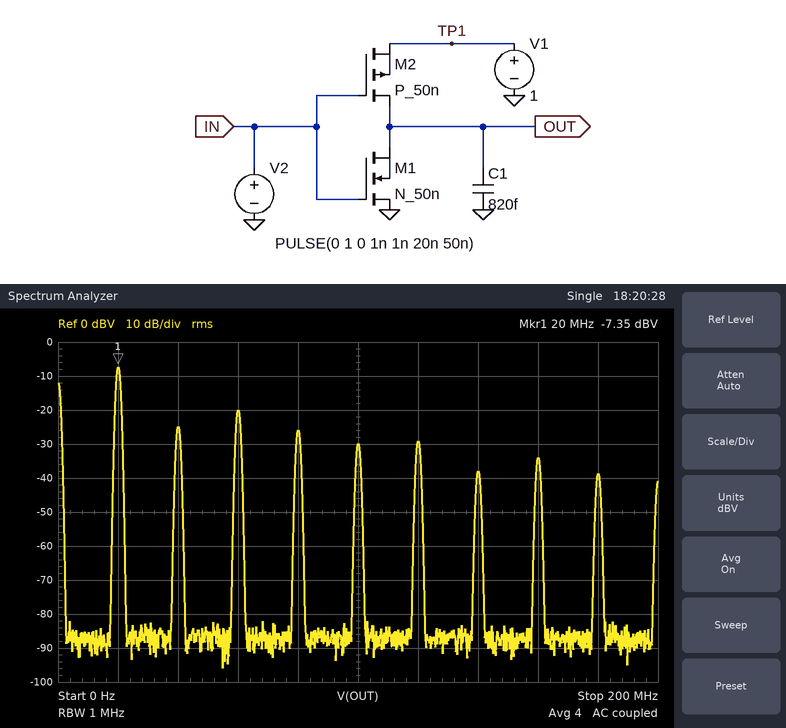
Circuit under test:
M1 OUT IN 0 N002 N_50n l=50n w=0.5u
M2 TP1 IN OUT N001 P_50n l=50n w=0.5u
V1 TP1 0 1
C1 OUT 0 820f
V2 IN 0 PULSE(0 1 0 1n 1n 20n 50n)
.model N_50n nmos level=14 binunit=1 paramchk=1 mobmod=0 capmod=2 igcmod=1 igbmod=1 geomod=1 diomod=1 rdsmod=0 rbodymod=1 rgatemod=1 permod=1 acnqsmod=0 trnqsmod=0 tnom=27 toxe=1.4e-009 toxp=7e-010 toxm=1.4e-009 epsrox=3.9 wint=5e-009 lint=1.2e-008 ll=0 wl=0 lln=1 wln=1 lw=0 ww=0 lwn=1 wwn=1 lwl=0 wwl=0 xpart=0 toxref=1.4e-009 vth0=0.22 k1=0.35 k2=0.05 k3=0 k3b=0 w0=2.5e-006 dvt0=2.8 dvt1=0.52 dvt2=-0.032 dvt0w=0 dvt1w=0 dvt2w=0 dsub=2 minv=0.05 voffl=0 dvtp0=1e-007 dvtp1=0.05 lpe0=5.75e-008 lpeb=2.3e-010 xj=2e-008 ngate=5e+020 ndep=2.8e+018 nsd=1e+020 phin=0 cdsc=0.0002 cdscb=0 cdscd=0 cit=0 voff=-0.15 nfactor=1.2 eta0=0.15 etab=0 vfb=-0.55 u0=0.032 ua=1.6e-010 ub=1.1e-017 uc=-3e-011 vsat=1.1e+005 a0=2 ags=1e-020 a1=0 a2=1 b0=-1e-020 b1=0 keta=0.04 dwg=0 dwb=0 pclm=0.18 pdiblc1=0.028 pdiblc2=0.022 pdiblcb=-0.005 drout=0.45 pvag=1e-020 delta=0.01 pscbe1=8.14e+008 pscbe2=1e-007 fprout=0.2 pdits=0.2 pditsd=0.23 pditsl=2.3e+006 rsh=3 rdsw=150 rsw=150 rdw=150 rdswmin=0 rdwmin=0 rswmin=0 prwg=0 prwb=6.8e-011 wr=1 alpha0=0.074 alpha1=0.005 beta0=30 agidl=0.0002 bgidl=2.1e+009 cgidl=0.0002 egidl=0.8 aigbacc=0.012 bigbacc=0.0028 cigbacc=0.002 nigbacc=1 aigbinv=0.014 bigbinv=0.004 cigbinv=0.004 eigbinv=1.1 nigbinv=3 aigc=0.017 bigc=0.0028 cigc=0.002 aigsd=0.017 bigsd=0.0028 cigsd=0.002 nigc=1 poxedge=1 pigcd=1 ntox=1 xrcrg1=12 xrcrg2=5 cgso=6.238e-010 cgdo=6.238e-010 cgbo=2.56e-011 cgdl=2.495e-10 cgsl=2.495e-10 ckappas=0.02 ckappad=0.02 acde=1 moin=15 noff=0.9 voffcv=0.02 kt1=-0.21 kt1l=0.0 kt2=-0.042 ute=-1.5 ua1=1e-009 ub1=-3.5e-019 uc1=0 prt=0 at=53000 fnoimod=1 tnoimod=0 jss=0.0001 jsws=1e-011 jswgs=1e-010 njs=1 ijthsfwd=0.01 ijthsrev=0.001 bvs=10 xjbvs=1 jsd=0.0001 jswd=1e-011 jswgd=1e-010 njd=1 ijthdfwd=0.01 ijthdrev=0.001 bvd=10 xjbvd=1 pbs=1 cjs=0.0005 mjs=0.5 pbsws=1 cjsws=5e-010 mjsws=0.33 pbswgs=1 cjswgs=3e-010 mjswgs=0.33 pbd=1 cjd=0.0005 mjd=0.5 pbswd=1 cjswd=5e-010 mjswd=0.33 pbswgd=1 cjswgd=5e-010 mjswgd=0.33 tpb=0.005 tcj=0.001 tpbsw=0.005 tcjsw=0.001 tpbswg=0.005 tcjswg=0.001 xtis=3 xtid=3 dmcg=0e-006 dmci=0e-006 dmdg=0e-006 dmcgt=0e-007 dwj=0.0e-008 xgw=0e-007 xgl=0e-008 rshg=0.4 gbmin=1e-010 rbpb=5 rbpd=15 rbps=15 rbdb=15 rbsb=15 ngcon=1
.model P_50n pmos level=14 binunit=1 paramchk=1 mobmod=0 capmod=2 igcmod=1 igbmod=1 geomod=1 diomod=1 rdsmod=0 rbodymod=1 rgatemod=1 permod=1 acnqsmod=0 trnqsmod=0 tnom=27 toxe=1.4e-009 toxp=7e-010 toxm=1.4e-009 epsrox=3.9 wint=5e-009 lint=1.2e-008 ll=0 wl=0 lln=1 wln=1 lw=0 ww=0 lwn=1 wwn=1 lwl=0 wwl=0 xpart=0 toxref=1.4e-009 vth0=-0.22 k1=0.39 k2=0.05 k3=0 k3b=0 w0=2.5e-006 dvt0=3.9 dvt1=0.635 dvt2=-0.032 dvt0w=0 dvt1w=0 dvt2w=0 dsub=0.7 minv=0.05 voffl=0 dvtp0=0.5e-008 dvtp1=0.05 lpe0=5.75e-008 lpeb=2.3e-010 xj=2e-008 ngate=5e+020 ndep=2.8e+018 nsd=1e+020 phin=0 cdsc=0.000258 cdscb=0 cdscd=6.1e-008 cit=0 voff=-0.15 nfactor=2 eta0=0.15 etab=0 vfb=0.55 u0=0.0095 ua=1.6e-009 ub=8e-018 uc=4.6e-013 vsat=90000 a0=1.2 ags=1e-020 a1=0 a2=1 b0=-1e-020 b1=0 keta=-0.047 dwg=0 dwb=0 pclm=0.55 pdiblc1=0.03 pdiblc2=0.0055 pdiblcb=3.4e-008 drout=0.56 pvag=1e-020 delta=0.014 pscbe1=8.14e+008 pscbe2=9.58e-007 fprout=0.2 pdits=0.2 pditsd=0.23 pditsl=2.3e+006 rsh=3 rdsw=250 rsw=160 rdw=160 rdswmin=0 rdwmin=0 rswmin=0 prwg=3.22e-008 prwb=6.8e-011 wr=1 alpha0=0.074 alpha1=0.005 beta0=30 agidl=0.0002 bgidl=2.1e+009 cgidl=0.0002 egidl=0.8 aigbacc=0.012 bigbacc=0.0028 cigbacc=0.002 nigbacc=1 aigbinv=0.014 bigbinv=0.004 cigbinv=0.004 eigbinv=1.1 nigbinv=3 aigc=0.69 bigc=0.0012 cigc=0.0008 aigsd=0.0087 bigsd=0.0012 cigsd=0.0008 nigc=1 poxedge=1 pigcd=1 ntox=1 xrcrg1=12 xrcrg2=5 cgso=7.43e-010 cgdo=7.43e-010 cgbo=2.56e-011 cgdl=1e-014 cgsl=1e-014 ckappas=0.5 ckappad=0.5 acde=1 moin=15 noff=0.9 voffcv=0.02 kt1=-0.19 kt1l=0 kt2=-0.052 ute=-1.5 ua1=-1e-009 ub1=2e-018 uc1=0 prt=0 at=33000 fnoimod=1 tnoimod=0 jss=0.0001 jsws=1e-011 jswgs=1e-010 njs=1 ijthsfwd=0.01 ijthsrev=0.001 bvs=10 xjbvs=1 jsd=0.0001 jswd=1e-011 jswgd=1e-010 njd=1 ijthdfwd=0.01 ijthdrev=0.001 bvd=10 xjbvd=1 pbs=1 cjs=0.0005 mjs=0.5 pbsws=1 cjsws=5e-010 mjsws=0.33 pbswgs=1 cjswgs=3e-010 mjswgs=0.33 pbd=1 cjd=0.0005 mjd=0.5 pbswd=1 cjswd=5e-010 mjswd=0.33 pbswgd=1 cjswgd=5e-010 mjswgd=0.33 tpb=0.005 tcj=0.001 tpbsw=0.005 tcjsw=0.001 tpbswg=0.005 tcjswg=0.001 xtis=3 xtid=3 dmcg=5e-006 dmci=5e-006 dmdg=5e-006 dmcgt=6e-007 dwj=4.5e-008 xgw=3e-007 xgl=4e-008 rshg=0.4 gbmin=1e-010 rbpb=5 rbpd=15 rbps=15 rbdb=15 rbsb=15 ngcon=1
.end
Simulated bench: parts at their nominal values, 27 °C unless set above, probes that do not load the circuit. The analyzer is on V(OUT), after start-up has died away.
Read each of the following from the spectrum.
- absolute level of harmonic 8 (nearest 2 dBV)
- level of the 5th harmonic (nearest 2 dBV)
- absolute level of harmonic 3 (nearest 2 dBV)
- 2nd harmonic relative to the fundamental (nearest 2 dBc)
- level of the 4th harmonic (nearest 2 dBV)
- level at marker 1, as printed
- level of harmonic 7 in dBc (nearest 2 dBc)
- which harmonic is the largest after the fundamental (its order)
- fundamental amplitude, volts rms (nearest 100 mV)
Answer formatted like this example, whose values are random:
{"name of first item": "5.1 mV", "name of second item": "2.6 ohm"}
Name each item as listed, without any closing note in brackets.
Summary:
{"absolute level of harmonic 8": "-34 dBV", "level of the 5th harmonic": "-30 dBV", "absolute level of harmonic 3": "-20 dBV", "2nd harmonic relative to the fundamental": "-18 dBc", "level of the 4th harmonic": "-26 dBV", "level at marker 1, as printed": "-7.35 dBV", "level of harmonic 7 in dBc": "-30 dBc", "which harmonic is the largest after the fundamental": "3", "fundamental amplitude, volts rms": "400 mV"}
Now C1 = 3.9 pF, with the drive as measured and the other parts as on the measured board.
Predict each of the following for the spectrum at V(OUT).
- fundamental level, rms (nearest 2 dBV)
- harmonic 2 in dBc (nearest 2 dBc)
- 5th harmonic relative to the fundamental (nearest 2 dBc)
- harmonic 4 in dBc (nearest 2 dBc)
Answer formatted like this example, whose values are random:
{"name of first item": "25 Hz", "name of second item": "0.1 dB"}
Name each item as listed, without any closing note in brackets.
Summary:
{"fundamental level, rms": "-12 dBV", "harmonic 2 in dBc": "-16 dBc", "5th harmonic relative to the fundamental": "-36 dBc", "harmonic 4 in dBc": "-26 dBc"}
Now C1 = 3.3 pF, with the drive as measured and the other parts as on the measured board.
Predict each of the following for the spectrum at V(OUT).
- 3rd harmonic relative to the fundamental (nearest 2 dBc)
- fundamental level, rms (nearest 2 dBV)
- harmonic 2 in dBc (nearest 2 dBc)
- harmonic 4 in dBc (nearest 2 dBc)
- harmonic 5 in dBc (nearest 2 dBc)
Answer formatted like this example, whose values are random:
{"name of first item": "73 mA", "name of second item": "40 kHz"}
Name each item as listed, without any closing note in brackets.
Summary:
{"3rd harmonic relative to the fundamental": "-20 dBc", "fundamental level, rms": "-10 dBV", "harmonic 2 in dBc": "-16 dBc", "harmonic 4 in dBc": "-24 dBc", "harmonic 5 in dBc": "-36 dBc"}
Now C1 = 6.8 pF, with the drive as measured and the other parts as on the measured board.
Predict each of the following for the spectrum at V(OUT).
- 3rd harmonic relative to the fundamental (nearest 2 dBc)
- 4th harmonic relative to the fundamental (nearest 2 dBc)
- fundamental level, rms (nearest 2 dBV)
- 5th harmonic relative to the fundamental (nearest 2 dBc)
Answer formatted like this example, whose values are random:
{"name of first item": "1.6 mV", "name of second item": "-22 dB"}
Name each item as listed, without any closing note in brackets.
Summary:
{"3rd harmonic relative to the fundamental": "-22 dBc", "4th harmonic relative to the fundamental": "-26 dBc", "fundamental level, rms": "-16 dBV", "5th harmonic relative to the fundamental": "-36 dBc"}
